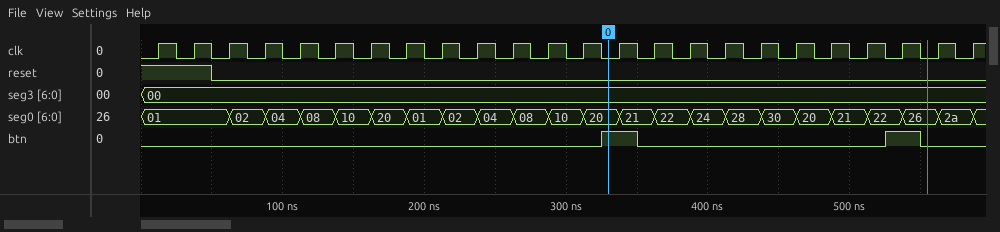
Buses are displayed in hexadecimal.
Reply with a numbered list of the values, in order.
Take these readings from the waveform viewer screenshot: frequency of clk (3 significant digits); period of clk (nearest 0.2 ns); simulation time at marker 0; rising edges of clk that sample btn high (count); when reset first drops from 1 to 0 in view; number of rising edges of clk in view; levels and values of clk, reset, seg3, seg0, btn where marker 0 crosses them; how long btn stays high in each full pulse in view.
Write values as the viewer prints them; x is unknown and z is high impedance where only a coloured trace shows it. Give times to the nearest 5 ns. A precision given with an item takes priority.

1. 40.0 MHz
2. 25 ns
3. 330 ns
4. 2
5. 50 ns
6. 24
7. clk=0, reset=0, seg3=00, seg0=20, btn=1
8. 25 ns, 25 ns
